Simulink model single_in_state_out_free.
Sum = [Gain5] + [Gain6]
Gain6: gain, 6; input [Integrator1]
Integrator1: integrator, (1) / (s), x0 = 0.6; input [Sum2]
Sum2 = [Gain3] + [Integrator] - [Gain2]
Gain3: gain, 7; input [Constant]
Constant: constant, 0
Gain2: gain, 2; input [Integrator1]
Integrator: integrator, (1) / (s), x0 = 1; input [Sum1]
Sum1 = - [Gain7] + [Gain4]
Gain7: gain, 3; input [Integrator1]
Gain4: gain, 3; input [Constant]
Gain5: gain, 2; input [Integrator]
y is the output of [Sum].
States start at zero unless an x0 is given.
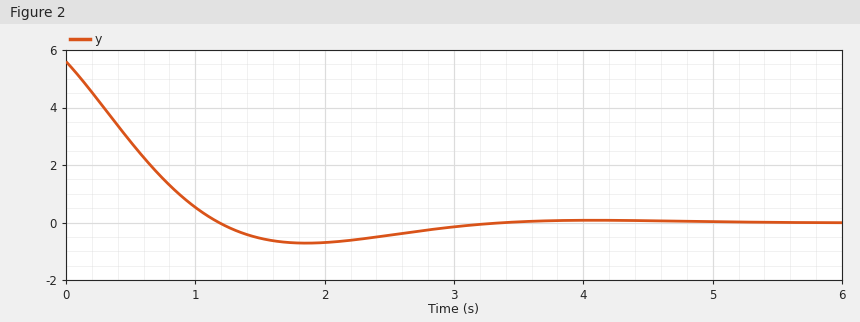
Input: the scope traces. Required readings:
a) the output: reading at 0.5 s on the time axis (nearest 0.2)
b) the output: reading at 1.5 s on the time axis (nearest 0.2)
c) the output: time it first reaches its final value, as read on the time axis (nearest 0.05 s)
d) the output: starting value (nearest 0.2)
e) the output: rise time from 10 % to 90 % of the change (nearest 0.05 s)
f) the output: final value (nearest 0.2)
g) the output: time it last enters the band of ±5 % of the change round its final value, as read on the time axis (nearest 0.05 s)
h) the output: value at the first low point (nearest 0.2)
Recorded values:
2.8
-0.6
1.20 s
5.6
0.90 s
0.0
2.75 s
-0.8
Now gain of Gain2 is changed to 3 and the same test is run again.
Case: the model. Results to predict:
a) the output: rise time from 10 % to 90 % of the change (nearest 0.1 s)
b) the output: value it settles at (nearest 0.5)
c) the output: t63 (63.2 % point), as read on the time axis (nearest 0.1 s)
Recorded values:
1.1 s
0.0
0.6 s
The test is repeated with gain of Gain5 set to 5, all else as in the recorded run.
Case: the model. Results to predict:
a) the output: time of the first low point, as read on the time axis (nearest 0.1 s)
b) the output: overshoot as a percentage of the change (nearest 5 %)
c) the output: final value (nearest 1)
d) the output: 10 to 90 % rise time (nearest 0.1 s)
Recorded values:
1.7 s
15 %
0
0.8 s
